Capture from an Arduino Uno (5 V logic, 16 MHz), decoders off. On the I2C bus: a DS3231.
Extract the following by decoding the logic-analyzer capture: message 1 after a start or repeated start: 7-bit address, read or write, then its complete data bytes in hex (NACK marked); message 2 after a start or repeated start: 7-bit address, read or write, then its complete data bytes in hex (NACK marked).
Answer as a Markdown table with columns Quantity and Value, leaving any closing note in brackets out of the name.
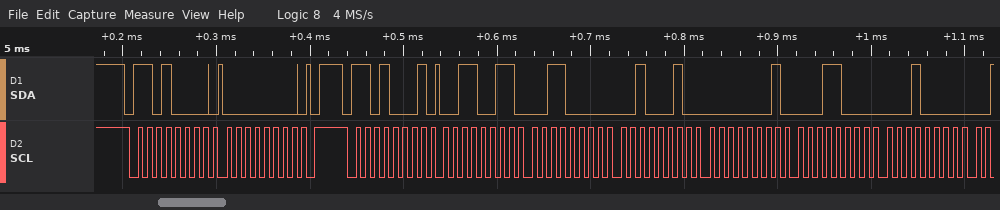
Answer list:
| Quantity | Value |
|---|---|
| message 1 after a start or repeated start: 7-bit address, read or write, then its complete data bytes in hex | 0x68 write: 00 |
| message 2 after a start or repeated start: 7-bit address, read or write, then its complete data bytes in hex | 0x68 read: 33 30 22 01 18 10 |
